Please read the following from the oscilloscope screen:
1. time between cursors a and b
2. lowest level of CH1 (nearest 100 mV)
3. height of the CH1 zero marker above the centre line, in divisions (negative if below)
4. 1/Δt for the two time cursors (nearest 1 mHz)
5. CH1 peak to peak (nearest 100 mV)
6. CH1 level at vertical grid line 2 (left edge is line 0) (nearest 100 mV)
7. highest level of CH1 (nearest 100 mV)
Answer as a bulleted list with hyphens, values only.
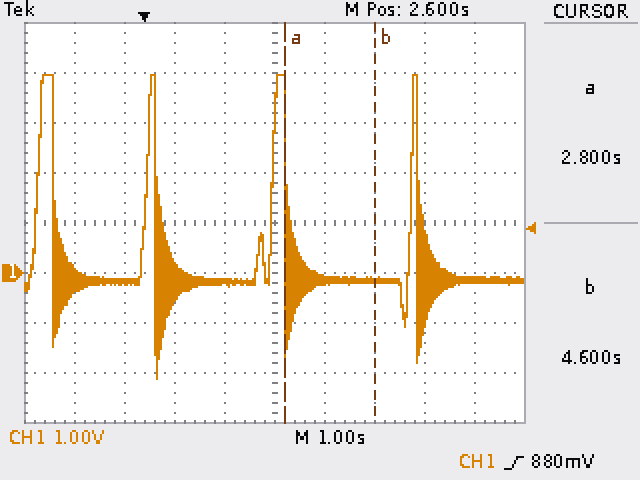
- 1.8 s
- -2.1 V
- -1.0 div
- 556 mHz
- 6.1 V
- -200 mV
- 4.0 V
